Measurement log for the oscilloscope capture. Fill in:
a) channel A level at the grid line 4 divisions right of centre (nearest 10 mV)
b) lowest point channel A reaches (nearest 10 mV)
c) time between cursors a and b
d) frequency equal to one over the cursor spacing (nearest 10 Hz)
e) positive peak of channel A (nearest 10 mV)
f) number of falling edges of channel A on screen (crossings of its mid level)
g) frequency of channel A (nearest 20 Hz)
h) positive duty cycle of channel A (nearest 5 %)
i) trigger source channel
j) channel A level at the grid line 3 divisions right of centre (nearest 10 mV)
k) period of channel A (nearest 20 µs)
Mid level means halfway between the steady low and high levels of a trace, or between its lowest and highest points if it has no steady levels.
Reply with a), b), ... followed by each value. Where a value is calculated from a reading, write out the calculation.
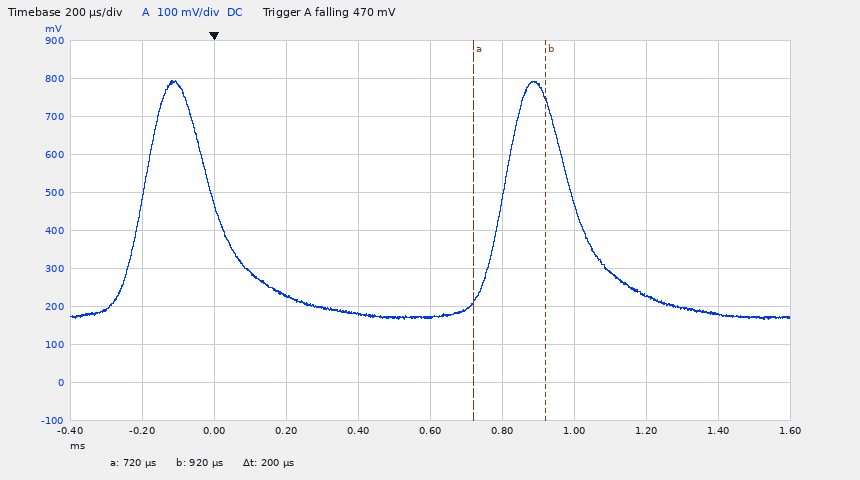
a) 180 mV
b) 170 mV
c) 200 µs
d) 1 / 200 µs ≈ 5.00 kHz
e) 790 mV
f) 2
g) 1 / 1.00 ms ≈ 1.00 kHz
h) 20 %
i) channel A
j) 230 mV
k) 1.00 ms
